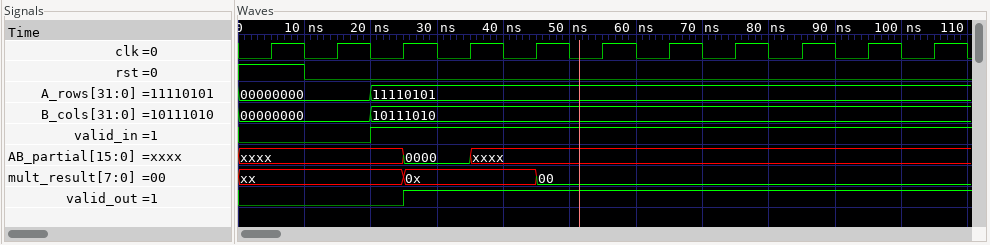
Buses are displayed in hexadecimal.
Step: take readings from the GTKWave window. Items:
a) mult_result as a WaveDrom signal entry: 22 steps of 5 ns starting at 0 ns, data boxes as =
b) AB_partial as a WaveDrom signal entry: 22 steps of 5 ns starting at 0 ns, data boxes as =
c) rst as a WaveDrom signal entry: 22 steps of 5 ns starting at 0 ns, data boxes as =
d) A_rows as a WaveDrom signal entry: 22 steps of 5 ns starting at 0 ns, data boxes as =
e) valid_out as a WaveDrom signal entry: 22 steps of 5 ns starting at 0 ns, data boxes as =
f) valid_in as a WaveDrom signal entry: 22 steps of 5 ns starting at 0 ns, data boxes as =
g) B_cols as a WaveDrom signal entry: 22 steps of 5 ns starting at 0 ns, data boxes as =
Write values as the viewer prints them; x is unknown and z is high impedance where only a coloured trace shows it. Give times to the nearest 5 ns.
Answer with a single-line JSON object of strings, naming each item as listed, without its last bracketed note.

{"mult_result as a WaveDrom signal entry: 22 steps of 5 ns starting at 0 ns, data boxes as =": "{name: 'mult_result', wave: 'x....=...=............', data: '0x 00'}", "AB_partial as a WaveDrom signal entry: 22 steps of 5 ns starting at 0 ns, data boxes as =": "{name: 'AB_partial', wave: 'x....=.x..............', data: '0000'}", "rst as a WaveDrom signal entry: 22 steps of 5 ns starting at 0 ns, data boxes as =": "{name: 'rst', wave: '1.0...................'}", "A_rows as a WaveDrom signal entry: 22 steps of 5 ns starting at 0 ns, data boxes as =": "{name: 'A_rows', wave: '=...=.................', data: '00000000 11110101'}", "valid_out as a WaveDrom signal entry: 22 steps of 5 ns starting at 0 ns, data boxes as =": "{name: 'valid_out', wave: '0....1................'}", "valid_in as a WaveDrom signal entry: 22 steps of 5 ns starting at 0 ns, data boxes as =": "{name: 'valid_in', wave: '0...1.................'}", "B_cols as a WaveDrom signal entry: 22 steps of 5 ns starting at 0 ns, data boxes as =": "{name: 'B_cols', wave: '=...=.................', data: '00000000 10111010'}"}
